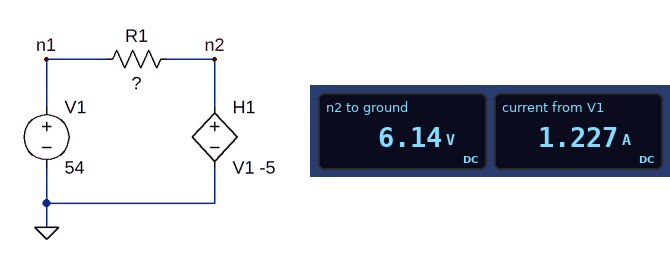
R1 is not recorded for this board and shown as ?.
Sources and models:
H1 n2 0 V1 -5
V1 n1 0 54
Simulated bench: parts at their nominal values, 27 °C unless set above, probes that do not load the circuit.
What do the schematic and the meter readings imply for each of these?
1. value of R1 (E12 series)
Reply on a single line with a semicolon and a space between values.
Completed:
39 Ω
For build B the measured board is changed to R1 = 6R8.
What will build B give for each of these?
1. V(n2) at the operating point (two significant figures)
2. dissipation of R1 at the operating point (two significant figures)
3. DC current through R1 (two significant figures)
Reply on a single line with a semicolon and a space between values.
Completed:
23 V; 140 W; 4.6 A
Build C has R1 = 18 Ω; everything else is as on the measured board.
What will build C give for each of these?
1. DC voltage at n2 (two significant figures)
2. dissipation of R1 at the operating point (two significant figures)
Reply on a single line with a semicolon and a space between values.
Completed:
12 V; 99 W
